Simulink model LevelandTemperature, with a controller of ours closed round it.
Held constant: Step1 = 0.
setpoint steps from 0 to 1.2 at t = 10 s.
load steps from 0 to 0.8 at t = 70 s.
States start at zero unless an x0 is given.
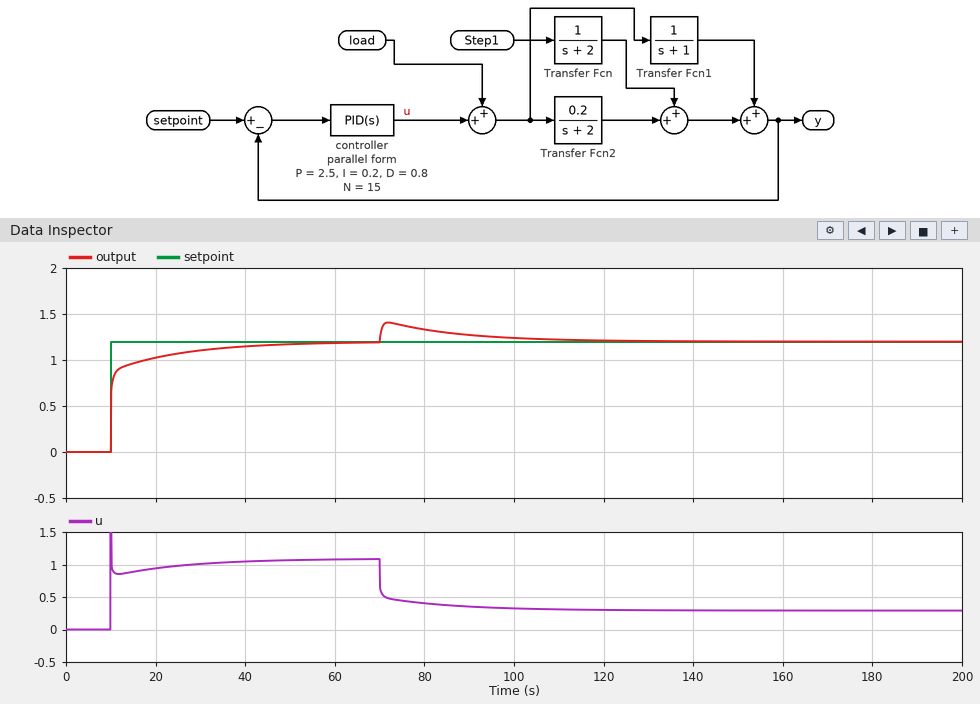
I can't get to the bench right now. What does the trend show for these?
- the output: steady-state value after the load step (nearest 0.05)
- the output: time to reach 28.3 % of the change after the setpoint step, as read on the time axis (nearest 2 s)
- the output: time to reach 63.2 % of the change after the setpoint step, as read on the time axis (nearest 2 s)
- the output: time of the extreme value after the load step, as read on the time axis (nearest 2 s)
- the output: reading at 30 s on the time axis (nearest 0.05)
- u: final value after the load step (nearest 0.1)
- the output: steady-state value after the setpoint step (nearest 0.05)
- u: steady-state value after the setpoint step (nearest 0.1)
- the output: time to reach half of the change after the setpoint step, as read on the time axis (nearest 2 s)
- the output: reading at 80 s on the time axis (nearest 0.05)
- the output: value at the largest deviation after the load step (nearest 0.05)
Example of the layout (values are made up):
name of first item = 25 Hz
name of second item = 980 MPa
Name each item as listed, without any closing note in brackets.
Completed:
the output: steady-state value after the load step = 1.20
the output: time to reach 28.3 % of the change after the setpoint step, as read on the time axis = 10 s
the output: time to reach 63.2 % of the change after the setpoint step, as read on the time axis = 10 s
the output: time of the extreme value after the load step, as read on the time axis = 72 s
the output: reading at 30 s on the time axis = 1.10
u: final value after the load step = 0.3
the output: steady-state value after the setpoint step = 1.20
u: steady-state value after the setpoint step = 1.1
the output: time to reach half of the change after the setpoint step, as read on the time axis = 10 s
the output: reading at 80 s on the time axis = 1.35
the output: value at the largest deviation after the load step = 1.40
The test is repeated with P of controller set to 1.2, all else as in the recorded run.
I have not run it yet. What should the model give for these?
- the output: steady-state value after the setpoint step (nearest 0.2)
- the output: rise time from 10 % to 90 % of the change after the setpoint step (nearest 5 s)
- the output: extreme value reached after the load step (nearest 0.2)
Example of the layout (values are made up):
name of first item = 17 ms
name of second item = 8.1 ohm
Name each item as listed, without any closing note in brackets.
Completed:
the output: steady-state value after the setpoint step = 1.2
the output: rise time from 10 % to 90 % of the change after the setpoint step = 15 s
the output: extreme value reached after the load step = 1.6
